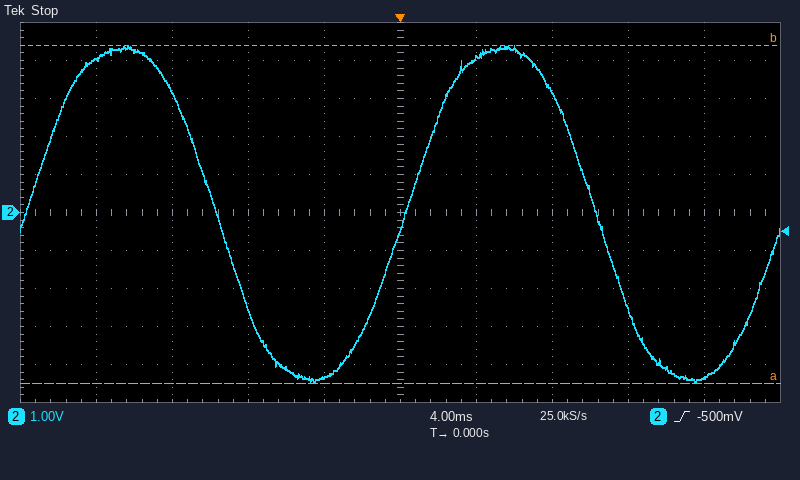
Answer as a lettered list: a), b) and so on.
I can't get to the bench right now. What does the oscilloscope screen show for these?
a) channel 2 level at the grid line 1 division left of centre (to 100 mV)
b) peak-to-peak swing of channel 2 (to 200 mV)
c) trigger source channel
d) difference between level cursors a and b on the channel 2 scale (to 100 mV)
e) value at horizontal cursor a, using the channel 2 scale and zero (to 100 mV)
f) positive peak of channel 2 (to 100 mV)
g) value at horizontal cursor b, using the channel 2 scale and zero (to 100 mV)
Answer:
a) -4.3 V
b) 8.8 V
c) channel 2
d) 8.9 V
e) -4.5 V
f) 4.4 V
g) 4.4 V
